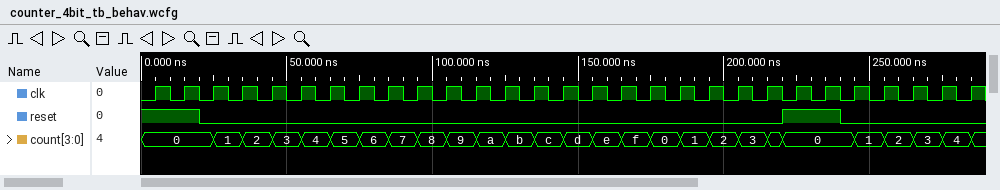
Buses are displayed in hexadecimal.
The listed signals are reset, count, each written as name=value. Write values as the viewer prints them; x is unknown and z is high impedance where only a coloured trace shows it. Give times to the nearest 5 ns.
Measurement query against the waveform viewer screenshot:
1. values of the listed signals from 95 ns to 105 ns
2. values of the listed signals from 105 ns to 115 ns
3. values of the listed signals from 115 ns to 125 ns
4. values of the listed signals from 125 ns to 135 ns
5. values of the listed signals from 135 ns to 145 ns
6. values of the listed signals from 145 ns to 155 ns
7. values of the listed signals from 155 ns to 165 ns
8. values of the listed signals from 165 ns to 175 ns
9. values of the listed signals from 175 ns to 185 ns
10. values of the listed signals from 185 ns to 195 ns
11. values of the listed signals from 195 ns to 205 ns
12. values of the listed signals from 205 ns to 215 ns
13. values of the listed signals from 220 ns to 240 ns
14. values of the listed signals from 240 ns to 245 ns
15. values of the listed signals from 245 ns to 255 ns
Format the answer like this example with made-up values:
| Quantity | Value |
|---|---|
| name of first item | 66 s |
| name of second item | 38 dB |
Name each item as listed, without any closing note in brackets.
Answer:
| Quantity | Value |
|---|---|
| values of the listed signals from 95 ns to 105 ns | reset=0, count=8 |
| values of the listed signals from 105 ns to 115 ns | reset=0, count=9 |
| values of the listed signals from 115 ns to 125 ns | reset=0, count=a |
| values of the listed signals from 125 ns to 135 ns | reset=0, count=b |
| values of the listed signals from 135 ns to 145 ns | reset=0, count=c |
| values of the listed signals from 145 ns to 155 ns | reset=0, count=d |
| values of the listed signals from 155 ns to 165 ns | reset=0, count=e |
| values of the listed signals from 165 ns to 175 ns | reset=0, count=f |
| values of the listed signals from 175 ns to 185 ns | reset=0, count=0 |
| values of the listed signals from 185 ns to 195 ns | reset=0, count=1 |
| values of the listed signals from 195 ns to 205 ns | reset=0, count=2 |
| values of the listed signals from 205 ns to 215 ns | reset=0, count=3 |
| values of the listed signals from 220 ns to 240 ns | reset=1, count=0 |
| values of the listed signals from 240 ns to 245 ns | reset=0, count=0 |
| values of the listed signals from 245 ns to 255 ns | reset=0, count=1 |
